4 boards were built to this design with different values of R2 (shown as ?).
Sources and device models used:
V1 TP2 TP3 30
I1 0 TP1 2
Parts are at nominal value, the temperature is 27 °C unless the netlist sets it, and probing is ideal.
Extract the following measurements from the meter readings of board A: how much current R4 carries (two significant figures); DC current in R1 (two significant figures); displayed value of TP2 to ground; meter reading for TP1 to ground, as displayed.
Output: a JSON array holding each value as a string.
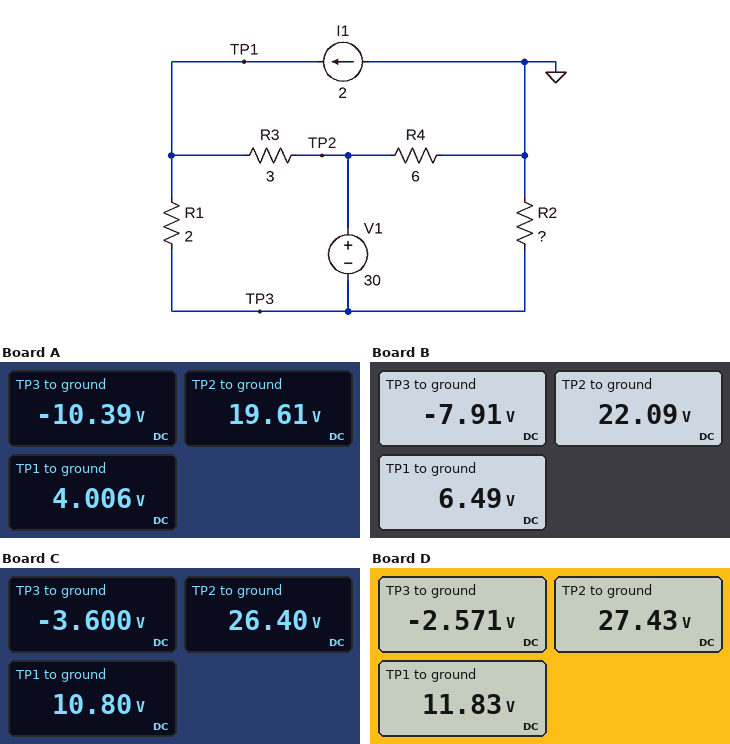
["3.3 A", "7.2 A", "19.61 V", "4.006 V"]
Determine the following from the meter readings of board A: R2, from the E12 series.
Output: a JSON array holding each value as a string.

["8.2 Ω"]
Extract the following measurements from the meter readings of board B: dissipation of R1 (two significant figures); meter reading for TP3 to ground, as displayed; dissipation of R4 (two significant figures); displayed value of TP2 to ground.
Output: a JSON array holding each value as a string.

["100 W", "-7.91 V", "81 W", "22.09 V"]
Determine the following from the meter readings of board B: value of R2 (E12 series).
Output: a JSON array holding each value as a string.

["4.7 Ω"]
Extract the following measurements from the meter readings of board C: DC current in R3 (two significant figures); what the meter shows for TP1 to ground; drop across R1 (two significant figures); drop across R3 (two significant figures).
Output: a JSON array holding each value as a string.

["5.2 A", "10.80 V", "14 V", "16 V"]
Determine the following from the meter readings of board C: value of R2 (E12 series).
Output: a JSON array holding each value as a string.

["1.5 Ω"]
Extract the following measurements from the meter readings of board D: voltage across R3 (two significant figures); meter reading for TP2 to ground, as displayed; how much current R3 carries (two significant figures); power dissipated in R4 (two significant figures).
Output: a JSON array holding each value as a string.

["16 V", "27.43 V", "5.2 A", "130 W"]
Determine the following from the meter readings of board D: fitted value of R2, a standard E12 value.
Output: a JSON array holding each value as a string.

["1 Ω"]
